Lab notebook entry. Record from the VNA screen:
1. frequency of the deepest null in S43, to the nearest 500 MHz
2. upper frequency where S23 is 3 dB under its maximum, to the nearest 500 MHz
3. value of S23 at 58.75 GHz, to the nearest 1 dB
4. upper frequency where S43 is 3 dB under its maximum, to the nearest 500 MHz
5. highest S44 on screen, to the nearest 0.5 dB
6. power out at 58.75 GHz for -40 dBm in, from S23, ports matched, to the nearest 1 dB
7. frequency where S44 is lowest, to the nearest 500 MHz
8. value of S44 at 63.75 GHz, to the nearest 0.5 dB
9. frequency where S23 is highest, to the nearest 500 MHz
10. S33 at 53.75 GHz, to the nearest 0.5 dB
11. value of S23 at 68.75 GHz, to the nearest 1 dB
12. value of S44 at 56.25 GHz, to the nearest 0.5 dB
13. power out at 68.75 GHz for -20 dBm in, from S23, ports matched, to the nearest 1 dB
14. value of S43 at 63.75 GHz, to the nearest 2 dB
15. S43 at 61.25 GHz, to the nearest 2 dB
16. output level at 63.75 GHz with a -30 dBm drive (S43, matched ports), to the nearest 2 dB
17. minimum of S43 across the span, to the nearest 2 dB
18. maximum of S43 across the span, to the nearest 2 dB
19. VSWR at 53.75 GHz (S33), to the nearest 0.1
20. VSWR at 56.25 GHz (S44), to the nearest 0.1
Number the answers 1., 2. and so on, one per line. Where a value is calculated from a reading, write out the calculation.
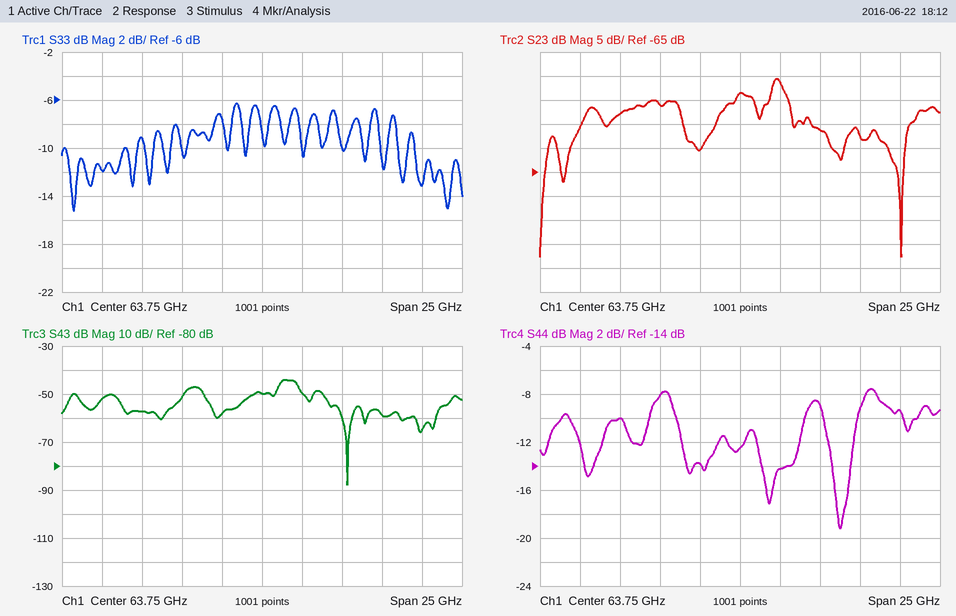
1. 69.0 GHz
2. 66.5 GHz
3. -51 dB
4. 66.0 GHz
5. -7.5 dB
6. -40 dBm + (-51 dB) = -91 dBm
7. 70.0 GHz
8. -12.5 dB
9. 66.0 GHz
10. -12.0 dB
11. -56 dB
12. -10.0 dB
13. -20 dBm + (-56 dB) = -76 dBm
14. -50 dB
15. -58 dB
16. -30 dBm + (-50 dB) = -80 dBm
17. -88 dB
18. -44 dB
19. |Γ| = 10^(-12/20) = 0.2512; VSWR = (1 + 0.2512)/(1 − 0.2512) ≈ 1.7
20. |Γ| = 10^(-10/20) = 0.3162; VSWR = (1 + 0.3162)/(1 − 0.3162) ≈ 1.9
